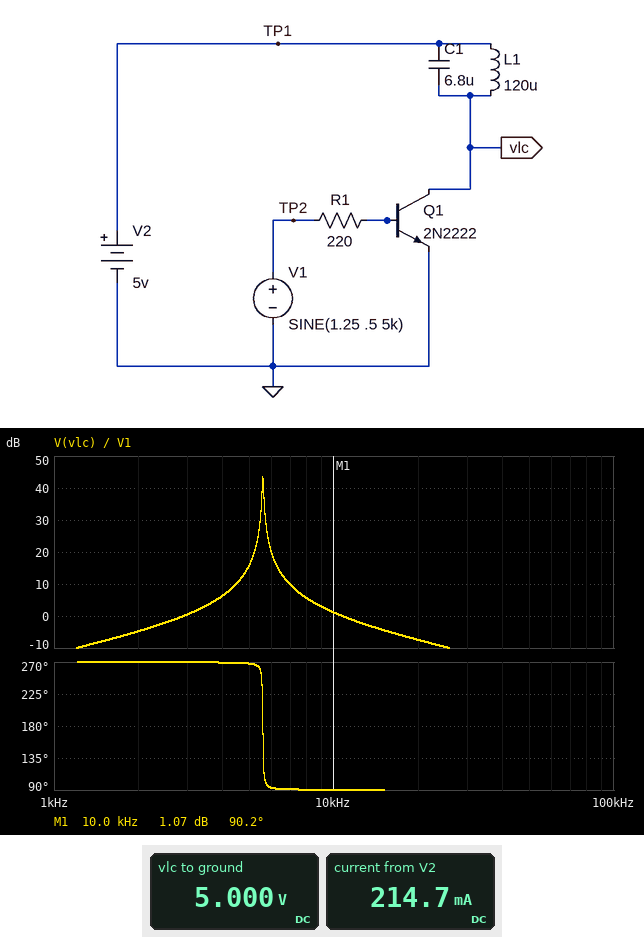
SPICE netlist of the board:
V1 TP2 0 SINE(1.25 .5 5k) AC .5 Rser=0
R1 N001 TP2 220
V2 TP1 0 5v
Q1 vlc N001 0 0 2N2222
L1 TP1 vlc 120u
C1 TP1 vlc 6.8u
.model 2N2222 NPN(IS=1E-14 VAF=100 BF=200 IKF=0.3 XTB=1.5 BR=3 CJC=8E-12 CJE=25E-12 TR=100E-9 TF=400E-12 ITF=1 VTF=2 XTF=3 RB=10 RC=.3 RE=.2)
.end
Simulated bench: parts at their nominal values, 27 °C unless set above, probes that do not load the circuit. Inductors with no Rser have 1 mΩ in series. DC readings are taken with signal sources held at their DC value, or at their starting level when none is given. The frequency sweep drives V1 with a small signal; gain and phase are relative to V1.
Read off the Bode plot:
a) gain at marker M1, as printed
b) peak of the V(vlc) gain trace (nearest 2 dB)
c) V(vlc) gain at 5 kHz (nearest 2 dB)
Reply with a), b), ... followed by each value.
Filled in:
a) 1.07 dB
b) 44 dB
c) 16 dB
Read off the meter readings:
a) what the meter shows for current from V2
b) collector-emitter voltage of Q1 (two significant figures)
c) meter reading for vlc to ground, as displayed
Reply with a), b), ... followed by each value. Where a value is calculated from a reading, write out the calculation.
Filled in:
a) 214.7 mA
b) 5 V = 5.0 V
c) 5.000 V
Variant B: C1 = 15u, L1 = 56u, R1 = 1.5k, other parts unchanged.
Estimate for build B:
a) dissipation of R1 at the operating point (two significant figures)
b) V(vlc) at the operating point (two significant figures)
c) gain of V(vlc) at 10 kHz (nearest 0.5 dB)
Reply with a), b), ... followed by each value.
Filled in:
a) 150 µW
b) 5.0 V
c) -17.0 dB
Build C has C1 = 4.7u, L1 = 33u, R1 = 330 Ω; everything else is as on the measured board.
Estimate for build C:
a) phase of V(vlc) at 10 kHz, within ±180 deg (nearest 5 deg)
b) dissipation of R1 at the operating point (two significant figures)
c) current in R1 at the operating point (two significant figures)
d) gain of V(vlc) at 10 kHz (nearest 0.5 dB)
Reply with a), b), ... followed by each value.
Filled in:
a) -90 deg
b) 500 µW
c) 1.2 mA
d) 3.0 dB
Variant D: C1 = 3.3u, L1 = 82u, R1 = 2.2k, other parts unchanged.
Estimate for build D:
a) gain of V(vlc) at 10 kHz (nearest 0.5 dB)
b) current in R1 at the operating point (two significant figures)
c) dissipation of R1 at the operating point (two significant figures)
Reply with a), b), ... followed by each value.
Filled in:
a) 14.5 dB
b) 220 µA
c) 110 µW
